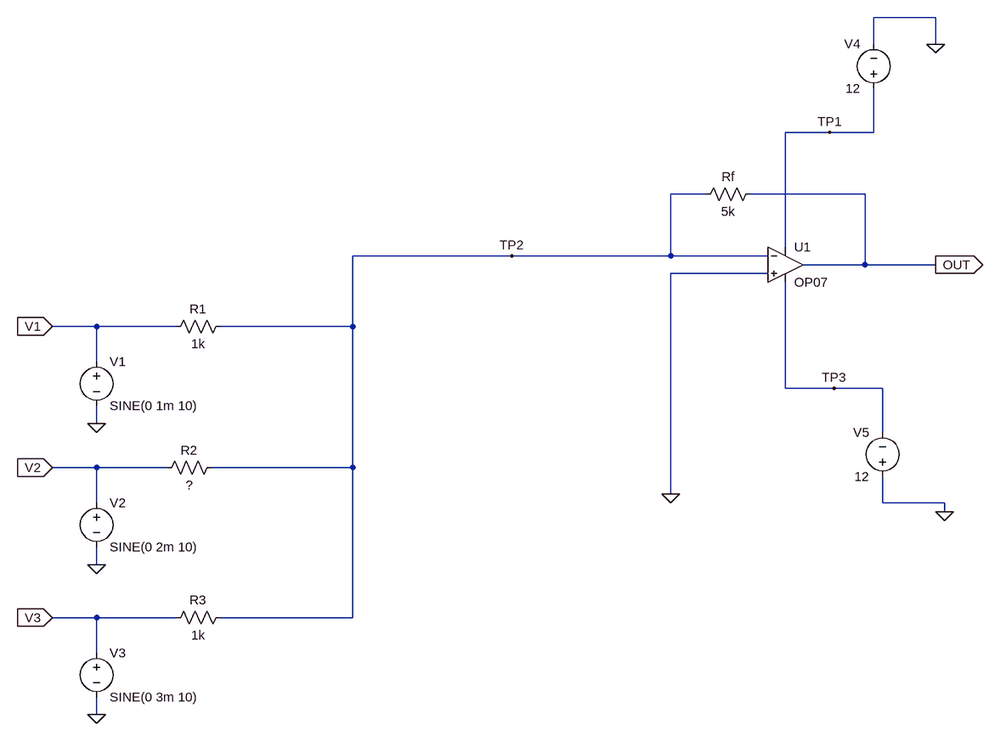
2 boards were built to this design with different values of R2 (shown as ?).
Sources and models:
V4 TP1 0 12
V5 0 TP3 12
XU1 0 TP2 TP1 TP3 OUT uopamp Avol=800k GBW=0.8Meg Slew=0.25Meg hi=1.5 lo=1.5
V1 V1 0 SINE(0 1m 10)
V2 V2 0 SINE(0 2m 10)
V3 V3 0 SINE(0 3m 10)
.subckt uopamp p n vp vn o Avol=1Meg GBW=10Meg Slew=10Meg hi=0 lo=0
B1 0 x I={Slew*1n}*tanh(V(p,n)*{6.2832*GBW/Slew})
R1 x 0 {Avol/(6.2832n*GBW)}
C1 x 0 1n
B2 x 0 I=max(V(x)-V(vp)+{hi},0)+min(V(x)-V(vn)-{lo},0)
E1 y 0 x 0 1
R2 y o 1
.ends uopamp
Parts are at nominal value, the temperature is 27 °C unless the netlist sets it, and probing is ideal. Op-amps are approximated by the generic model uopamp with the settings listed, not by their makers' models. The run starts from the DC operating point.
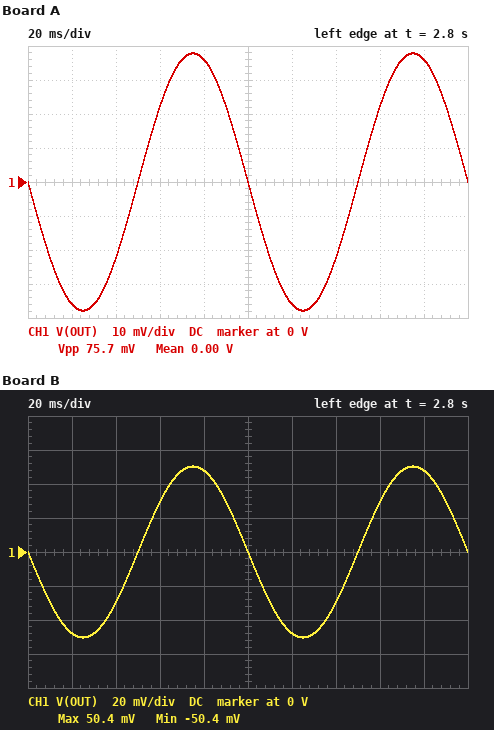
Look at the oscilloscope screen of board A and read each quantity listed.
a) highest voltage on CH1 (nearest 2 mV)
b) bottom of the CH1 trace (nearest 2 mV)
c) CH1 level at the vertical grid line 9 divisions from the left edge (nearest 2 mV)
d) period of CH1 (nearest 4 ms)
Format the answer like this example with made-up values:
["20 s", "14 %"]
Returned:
["38 mV", "-38 mV", "36 mV", "100 ms"]
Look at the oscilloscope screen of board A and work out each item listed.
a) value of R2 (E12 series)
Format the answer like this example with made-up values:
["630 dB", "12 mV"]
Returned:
["560 Ω"]
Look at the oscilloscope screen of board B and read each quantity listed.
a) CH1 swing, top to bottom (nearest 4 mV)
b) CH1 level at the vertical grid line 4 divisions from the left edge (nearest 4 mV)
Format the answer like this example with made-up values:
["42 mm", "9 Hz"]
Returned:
["100 mV", "48 mV"]
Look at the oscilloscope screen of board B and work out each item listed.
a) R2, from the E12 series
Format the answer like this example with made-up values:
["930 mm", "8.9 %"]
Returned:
["330 Ω"]
